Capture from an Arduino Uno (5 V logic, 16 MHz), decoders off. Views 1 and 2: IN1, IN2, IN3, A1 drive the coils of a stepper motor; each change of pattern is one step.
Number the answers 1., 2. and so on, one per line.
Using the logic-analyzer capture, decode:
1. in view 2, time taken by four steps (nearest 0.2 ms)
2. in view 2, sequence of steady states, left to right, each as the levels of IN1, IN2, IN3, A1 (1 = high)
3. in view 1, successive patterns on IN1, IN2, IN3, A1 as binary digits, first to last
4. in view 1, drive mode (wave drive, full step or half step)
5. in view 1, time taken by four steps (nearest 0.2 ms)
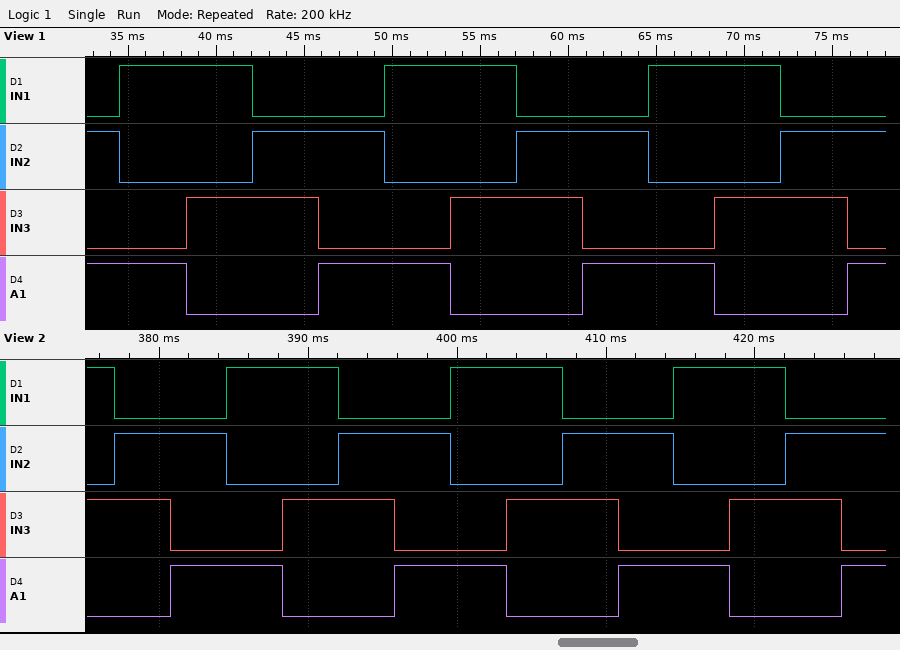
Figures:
1. 15.0 ms
2. 1010 0110 0101 1001 1010 0110 0101 1001 1010 0110 0101 1001 1010 0110 0101
3. 0101 1001 1010 0110 0101 1001 1010 0110 0101 1001 1010 0110 0101
4. full step
5. 15.0 ms
